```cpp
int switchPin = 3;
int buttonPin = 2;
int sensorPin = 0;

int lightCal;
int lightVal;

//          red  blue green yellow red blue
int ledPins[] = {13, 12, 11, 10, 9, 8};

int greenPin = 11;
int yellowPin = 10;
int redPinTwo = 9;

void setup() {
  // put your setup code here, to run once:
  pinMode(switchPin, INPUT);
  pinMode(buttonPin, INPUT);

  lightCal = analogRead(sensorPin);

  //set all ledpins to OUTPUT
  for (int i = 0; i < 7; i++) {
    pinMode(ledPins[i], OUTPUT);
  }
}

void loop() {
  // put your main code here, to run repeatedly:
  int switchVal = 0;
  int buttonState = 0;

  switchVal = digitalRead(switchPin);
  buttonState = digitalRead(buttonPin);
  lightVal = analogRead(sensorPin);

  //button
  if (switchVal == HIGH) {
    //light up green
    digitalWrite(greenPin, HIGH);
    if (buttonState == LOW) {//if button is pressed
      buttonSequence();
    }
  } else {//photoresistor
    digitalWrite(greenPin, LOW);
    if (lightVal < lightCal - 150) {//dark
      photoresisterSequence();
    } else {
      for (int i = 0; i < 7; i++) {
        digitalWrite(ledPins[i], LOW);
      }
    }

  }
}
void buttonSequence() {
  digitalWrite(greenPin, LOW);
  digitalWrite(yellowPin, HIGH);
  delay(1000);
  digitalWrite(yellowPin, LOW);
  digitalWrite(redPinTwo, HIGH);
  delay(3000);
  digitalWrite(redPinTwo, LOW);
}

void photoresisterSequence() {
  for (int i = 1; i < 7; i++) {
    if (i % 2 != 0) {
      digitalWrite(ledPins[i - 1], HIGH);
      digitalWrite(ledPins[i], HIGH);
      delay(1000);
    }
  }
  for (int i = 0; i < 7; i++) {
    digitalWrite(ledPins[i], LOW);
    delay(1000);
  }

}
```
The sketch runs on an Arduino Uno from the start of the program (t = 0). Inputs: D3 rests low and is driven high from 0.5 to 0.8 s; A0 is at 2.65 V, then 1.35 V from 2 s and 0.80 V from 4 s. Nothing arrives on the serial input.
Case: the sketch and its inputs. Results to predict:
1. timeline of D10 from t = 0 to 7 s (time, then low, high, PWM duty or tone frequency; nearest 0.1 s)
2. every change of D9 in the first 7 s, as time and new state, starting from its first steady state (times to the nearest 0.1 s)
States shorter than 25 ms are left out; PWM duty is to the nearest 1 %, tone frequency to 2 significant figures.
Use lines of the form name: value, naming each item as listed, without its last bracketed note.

timeline of D10 from t = 0 to 7 s: 0 s low; 0.5 s high; 1.5 s low; 5.5 s high
every change of D9 in the first 7 s, as time and new state, starting from its first steady state: 0 s low; 1.5 s high; 4.5 s low; 6.5 s high
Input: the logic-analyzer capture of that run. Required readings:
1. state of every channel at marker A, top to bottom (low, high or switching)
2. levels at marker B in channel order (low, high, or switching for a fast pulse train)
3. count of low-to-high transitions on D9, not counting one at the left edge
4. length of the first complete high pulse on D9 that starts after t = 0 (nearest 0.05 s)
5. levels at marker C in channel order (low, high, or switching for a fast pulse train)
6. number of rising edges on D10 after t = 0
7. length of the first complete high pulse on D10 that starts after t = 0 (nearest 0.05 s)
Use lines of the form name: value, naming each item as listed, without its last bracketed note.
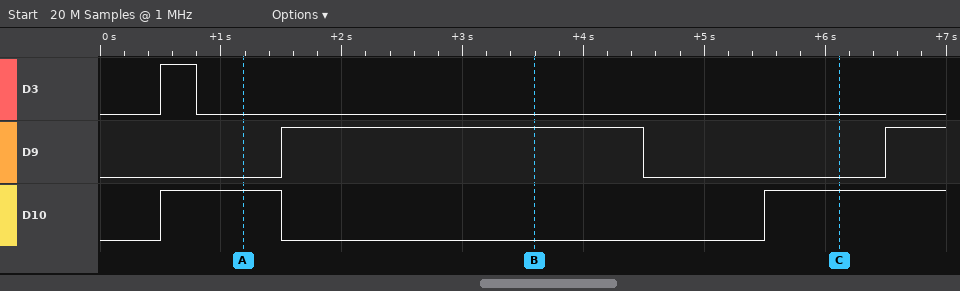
state of every channel at marker A, top to bottom: D3 low, D9 low, D10 high
levels at marker B in channel order: D3 low, D9 high, D10 low
count of low-to-high transitions on D9, not counting one at the left edge: 2
length of the first complete high pulse on D9 that starts after t = 0: 3.00 s
levels at marker C in channel order: D3 low, D9 low, D10 high
number of rising edges on D10 after t = 0: 2
length of the first complete high pulse on D10 that starts after t = 0: 1.00 s
